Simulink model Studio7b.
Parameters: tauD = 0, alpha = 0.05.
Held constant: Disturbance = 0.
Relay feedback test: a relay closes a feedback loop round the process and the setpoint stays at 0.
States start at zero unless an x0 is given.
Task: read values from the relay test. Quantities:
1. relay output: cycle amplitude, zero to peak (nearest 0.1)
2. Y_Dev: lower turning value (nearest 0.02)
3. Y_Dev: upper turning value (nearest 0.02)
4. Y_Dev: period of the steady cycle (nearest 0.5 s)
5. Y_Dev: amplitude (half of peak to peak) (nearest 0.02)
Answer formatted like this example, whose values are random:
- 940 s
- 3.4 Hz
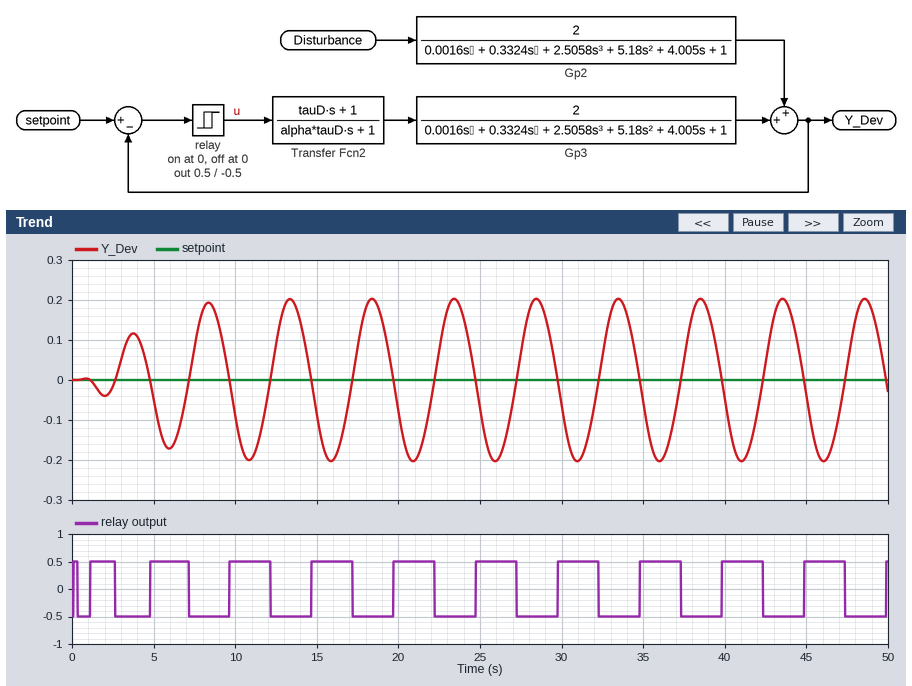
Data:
- 0.5
- -0.20
- 0.20
- 5.0 s
- 0.20
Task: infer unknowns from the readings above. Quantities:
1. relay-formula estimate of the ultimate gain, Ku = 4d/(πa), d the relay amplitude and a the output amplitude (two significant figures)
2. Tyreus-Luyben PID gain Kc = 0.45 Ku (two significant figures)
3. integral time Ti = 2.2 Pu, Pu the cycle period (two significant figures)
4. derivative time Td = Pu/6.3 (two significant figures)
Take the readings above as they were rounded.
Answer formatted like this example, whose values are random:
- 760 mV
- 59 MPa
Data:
- 3.2
- 1.4
- 11 s
- 0.79 s
